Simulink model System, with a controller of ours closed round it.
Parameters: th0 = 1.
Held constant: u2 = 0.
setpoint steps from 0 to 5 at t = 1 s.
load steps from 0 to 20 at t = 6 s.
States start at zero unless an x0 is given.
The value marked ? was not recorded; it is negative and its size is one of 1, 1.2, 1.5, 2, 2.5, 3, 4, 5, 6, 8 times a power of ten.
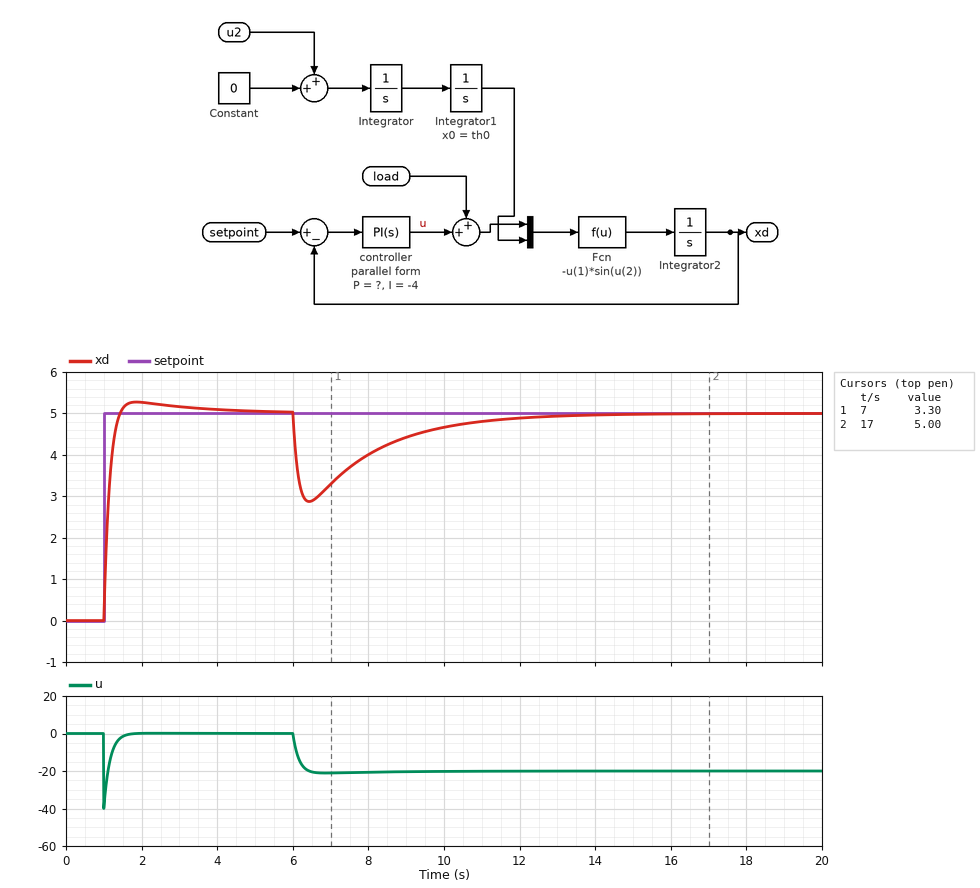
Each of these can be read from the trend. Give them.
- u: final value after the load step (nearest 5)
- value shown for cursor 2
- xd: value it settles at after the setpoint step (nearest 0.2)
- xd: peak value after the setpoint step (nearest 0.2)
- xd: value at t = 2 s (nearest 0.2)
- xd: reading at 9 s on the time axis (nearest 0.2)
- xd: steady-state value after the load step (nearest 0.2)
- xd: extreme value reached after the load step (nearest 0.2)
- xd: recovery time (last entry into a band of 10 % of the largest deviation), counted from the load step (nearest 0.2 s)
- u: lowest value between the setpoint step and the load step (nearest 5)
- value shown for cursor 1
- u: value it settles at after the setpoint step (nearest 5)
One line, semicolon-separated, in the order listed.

-20; 5.00; 5.0; 5.2; 5.2; 4.4; 5.0; 2.8; 4.8 s; -40; 3.30; 0
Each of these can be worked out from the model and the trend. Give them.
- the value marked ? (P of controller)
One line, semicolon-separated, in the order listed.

-8
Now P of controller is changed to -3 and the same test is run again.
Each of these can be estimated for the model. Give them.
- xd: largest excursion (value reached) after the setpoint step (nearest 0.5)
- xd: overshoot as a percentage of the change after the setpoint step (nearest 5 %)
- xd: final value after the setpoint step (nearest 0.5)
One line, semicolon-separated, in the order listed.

6.0; 20 %; 5.0
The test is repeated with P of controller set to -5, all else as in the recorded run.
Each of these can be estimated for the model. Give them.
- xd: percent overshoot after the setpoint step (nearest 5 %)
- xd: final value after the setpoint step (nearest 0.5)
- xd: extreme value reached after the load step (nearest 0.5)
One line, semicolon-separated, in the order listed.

10 %; 5.0; 2.0
